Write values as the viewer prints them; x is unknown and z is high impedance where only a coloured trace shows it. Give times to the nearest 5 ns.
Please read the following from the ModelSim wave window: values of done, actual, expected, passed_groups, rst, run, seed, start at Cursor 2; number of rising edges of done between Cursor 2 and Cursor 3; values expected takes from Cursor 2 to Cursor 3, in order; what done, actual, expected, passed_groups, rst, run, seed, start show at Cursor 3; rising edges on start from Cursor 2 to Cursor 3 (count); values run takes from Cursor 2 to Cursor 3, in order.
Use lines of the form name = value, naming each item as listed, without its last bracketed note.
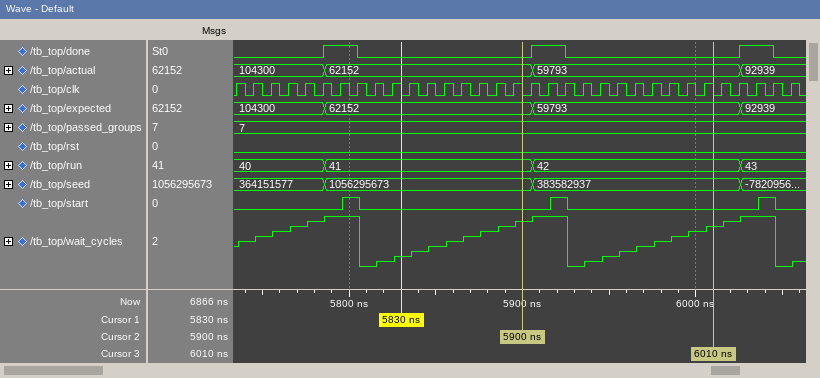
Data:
values of done, actual, expected, passed_groups, rst, run, seed, start at Cursor 2 = done=0, actual=62152, expected=62152, passed_groups=7, rst=0, run=41, seed=1056295673, start=0
number of rising edges of done between Cursor 2 and Cursor 3 = 1
values expected takes from Cursor 2 to Cursor 3, in order = 62152, 59793
what done, actual, expected, passed_groups, rst, run, seed, start show at Cursor 3 = done=0, actual=59793, expected=59793, passed_groups=7, rst=0, run=42, seed=383582937, start=0
rising edges on start from Cursor 2 to Cursor 3 = 1
values run takes from Cursor 2 to Cursor 3, in order = 41, 42
